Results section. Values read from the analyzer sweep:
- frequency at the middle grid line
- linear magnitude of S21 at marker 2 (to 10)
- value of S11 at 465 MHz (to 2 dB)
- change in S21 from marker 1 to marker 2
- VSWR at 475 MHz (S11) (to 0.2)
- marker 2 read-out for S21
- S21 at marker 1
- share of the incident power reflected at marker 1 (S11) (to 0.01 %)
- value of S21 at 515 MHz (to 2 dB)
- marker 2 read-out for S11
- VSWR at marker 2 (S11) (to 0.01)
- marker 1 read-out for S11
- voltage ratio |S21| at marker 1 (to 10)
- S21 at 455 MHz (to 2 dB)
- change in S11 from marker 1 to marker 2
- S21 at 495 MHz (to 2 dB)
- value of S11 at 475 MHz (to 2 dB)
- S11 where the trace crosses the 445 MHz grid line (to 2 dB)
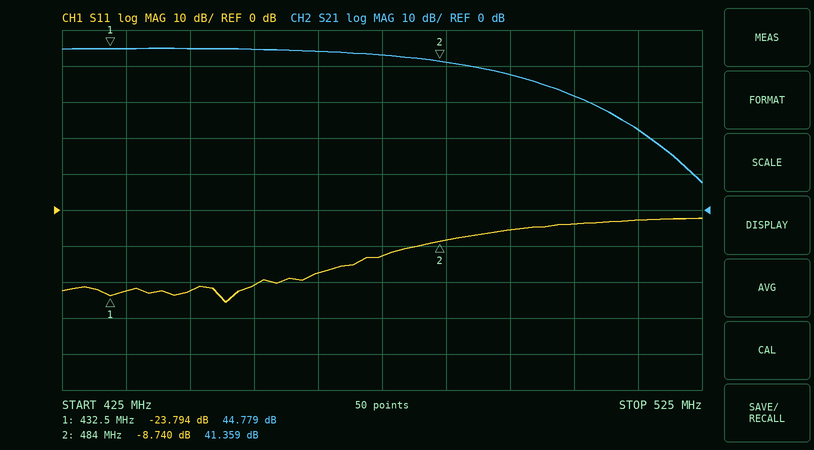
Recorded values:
475 MHz
120
-18 dB
-3.420 dB
1.6
41.359 dB
44.779 dB
0.42 %
22 dB
-8.740 dB
2.15
-23.794 dB
170
44 dB
15.054 dB
38 dB
-12 dB
-22 dB
